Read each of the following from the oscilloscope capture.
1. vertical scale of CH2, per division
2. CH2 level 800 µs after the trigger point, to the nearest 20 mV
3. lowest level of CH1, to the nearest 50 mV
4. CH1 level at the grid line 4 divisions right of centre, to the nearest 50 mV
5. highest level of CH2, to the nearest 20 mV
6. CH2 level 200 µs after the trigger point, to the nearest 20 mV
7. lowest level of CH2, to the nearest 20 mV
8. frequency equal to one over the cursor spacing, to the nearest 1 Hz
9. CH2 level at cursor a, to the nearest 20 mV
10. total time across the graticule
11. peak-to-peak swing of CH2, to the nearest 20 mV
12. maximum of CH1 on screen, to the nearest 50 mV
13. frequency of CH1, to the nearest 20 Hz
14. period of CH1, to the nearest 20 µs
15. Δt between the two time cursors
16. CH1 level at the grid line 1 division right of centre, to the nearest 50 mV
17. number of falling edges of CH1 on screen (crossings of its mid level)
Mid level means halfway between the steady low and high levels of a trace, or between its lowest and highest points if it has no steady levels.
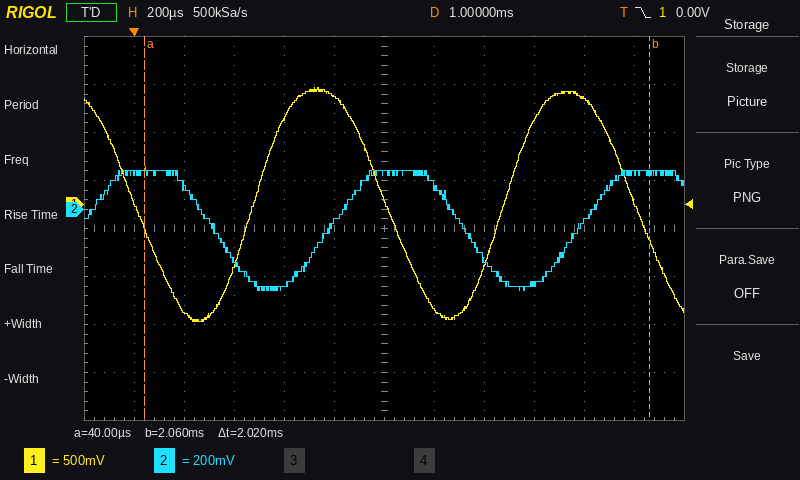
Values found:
200 mV
-60 mV
-1.20 V
1.10 V
180 mV
100 mV
-340 mV
495 Hz
160 mV
2.4 ms
520 mV
1.20 V
1.00 kHz
1.00 ms
2.02 ms
-1.10 V
3
